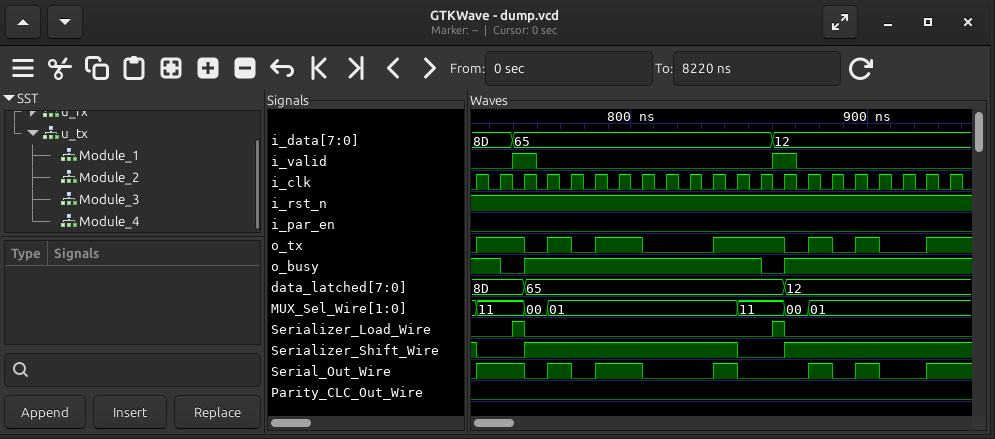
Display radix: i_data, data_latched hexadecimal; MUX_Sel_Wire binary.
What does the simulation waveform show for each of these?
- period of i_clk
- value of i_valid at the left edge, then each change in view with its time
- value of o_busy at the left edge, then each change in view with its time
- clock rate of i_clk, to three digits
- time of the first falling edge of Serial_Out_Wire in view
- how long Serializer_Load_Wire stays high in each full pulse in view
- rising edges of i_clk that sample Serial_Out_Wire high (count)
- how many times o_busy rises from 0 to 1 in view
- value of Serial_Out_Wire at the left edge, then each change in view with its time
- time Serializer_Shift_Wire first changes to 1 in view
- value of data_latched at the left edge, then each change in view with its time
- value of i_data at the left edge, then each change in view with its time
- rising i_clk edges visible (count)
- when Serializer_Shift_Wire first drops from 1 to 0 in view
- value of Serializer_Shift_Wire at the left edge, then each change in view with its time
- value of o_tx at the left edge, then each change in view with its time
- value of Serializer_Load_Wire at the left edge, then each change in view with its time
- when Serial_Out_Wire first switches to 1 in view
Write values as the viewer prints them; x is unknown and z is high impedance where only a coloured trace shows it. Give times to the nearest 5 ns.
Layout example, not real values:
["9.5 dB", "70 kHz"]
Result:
["10 ns", "0, 1 at 750 ns, 0 at 760 ns, 1 at 860 ns, 0 at 870 ns", "1, 0 at 745 ns, 1 at 755 ns, 0 at 855 ns, 1 at 865 ns", "100 MHz", "755 ns", "5 ns, 5 ns", "9", "2", "0, 1 at 735 ns, 0 at 755 ns, 1 at 765 ns, 0 at 775 ns, 1 at 785 ns, 0 at 805 ns, 1 at 835 ns, 0 at 845 ns, 1 at 875 ns, 0 at 885 ns, 1 at 895 ns, 0 at 905 ns, 1 at 925 ns", "755 ns", "8D, 65 at 755 ns, 12 at 865 ns", "8D, 65 at 750 ns, 12 at 860 ns", "21", "735 ns", "1, 0 at 735 ns, 1 at 755 ns, 0 at 845 ns, 1 at 865 ns", "0, 1 at 735 ns, 0 at 755 ns, 1 at 765 ns, 0 at 775 ns, 1 at 785 ns, 0 at 805 ns, 1 at 835 ns, 0 at 865 ns, 1 at 875 ns, 0 at 885 ns, 1 at 895 ns, 0 at 905 ns, 1 at 925 ns", "0, 1 at 750 ns, 0 at 755 ns, 1 at 860 ns, 0 at 865 ns", "735 ns"]
